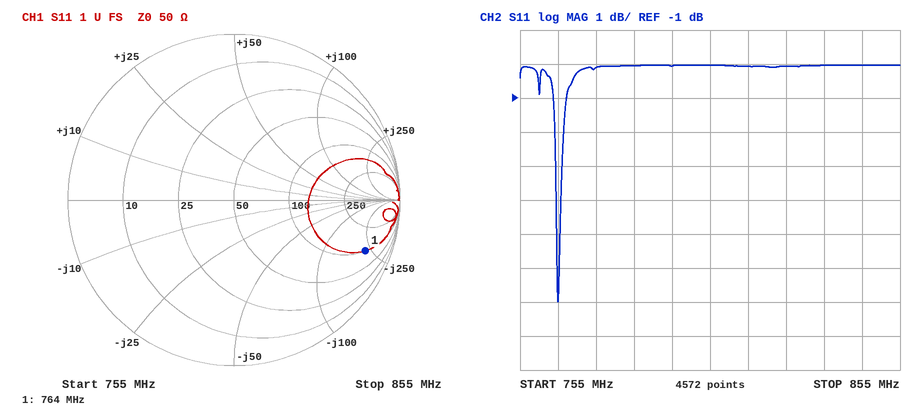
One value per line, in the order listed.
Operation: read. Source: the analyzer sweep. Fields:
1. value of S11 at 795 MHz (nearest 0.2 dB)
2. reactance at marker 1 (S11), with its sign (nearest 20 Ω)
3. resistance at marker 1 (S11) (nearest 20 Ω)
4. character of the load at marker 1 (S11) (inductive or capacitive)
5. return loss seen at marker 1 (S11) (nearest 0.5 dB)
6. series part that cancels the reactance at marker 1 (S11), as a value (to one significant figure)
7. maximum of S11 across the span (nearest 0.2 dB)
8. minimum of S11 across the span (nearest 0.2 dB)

0.0 dB
-220 Ω
100 Ω
capacitive
1.5 dB
50 nH
0.0 dB
-7.0 dB
